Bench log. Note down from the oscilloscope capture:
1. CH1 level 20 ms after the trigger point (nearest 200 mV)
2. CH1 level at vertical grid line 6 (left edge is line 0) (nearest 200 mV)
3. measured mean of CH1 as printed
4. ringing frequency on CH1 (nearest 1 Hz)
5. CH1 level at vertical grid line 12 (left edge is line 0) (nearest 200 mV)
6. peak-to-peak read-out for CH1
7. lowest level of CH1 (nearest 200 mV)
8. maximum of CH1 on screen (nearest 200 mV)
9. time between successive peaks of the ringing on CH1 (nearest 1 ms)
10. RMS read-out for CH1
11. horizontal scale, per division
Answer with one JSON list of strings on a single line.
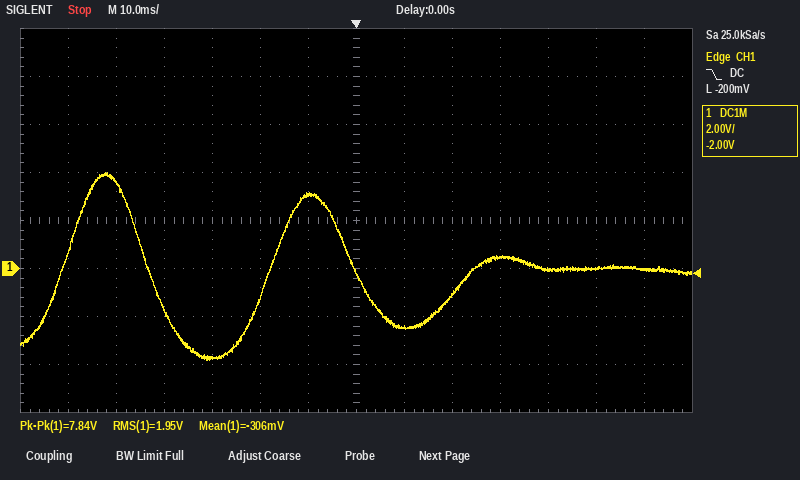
["-1.0 V", "3.0 V", "-306 mV", "24 Hz", "0.0 V", "7.84 V", "-3.8 V", "4.0 V", "41 ms", "1.95 V", "10 ms"]
